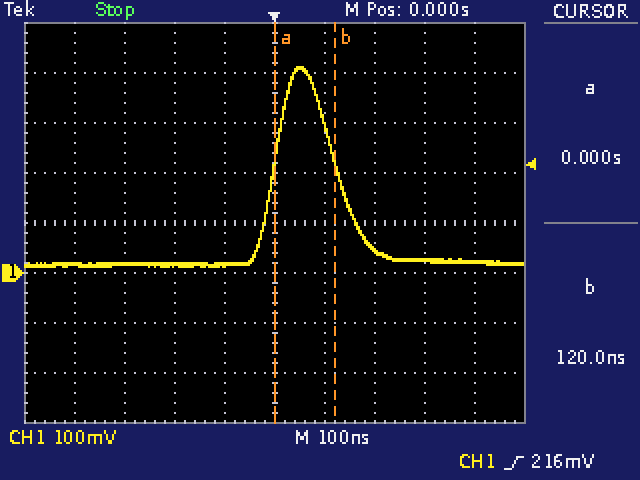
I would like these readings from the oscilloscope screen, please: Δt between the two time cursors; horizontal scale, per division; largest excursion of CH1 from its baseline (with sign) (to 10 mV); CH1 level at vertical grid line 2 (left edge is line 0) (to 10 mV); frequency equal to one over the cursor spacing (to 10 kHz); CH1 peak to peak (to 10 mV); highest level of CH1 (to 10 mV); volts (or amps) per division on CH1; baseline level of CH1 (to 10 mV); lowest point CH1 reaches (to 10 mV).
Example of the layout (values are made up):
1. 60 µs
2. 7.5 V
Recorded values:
1. 120 ns
2. 100 ns
3. +390 mV
4. 20 mV
5. 8.33 MHz
6. 400 mV
7. 410 mV
8. 100 mV
9. 20 mV
10. 10 mV
